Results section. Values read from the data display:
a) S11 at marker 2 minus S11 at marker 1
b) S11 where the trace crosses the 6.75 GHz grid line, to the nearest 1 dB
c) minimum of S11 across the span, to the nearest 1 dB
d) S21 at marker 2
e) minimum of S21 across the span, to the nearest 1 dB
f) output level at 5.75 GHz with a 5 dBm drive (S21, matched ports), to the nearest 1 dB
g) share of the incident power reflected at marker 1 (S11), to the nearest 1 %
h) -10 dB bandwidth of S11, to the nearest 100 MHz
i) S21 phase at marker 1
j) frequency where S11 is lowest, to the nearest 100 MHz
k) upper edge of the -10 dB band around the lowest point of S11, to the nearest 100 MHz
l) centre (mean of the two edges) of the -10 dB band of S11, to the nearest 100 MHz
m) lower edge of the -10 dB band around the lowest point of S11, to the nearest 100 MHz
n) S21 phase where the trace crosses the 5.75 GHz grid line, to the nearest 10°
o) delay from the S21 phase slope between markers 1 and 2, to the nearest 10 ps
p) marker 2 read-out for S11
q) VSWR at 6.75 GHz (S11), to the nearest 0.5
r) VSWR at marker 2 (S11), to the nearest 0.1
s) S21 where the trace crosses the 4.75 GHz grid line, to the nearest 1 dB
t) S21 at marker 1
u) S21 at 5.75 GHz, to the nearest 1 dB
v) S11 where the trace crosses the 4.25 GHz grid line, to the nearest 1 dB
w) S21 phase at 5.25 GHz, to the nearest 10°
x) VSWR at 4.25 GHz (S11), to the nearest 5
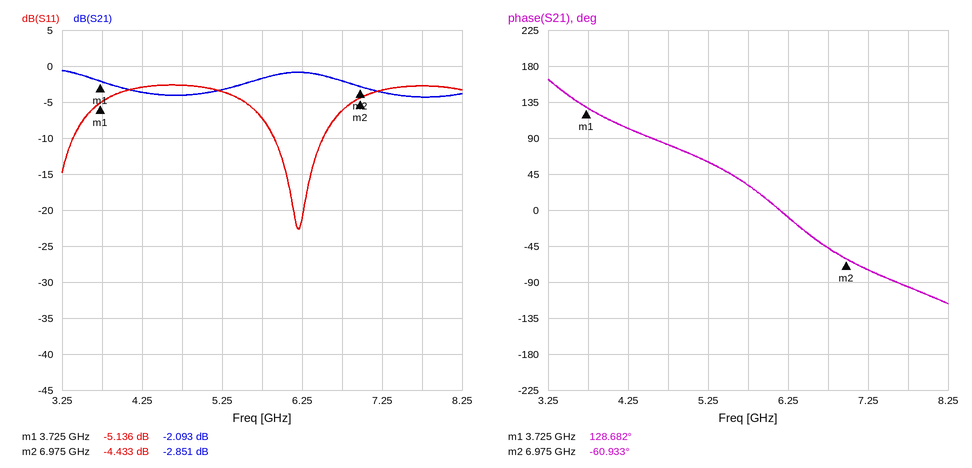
0.703 dB
-6 dB
-23 dB
-2.851 dB
-4 dB
3 dBm
31 %
600 MHz
128.682°
6.2 GHz
6.5 GHz
6.2 GHz
5.9 GHz
30°
160 ps
-4.433 dB
3.0
4.0
-4 dB
-2.093 dB
-2 dB
-3 dB
60°
5
